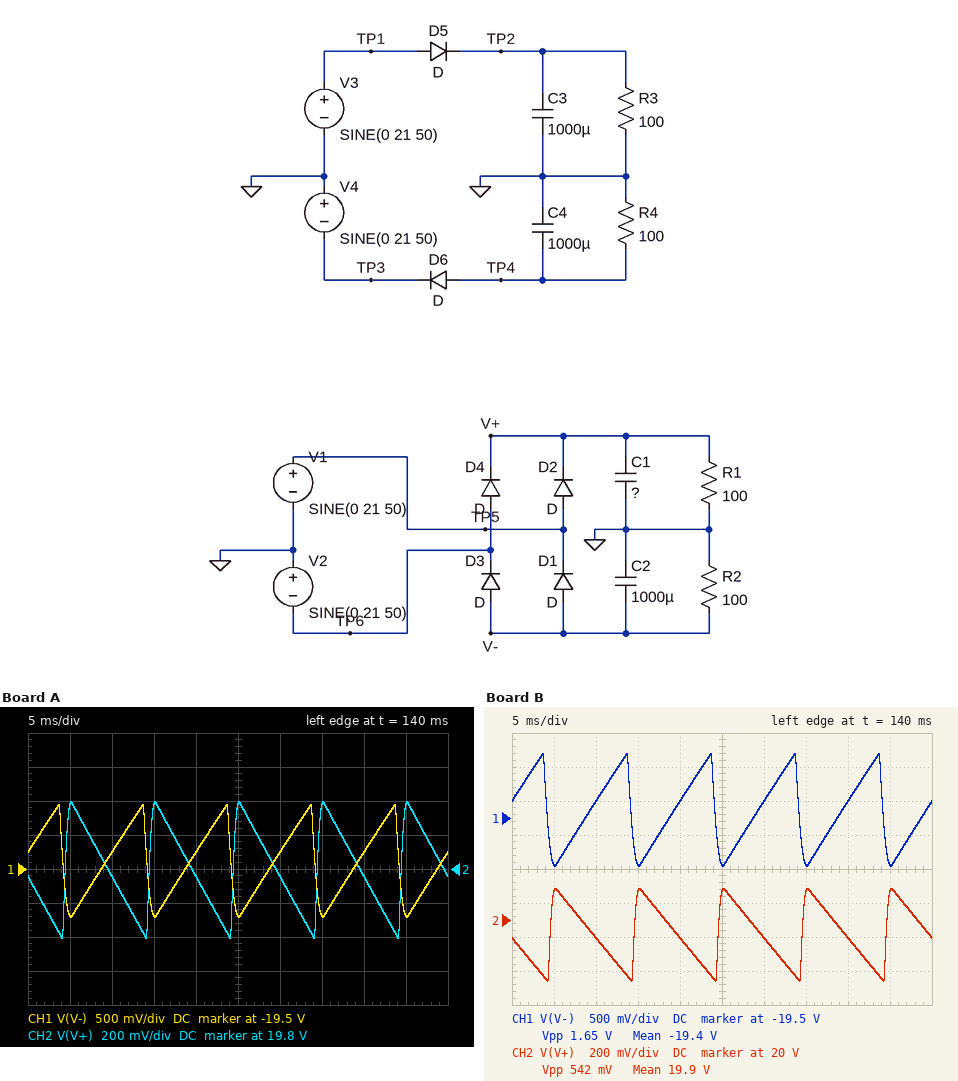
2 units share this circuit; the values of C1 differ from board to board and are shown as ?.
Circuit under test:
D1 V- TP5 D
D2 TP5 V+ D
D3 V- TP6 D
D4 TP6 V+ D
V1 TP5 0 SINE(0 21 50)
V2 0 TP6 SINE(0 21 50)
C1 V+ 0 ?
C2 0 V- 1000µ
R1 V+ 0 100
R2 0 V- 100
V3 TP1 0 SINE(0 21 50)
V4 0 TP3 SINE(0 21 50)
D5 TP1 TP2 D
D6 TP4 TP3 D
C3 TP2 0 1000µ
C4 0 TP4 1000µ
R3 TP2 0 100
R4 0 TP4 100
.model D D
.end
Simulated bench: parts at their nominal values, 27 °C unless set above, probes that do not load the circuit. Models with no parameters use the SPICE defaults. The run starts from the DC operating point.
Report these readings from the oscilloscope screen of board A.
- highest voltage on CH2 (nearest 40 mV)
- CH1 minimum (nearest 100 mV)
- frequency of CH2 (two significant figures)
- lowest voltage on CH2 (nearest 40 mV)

20.20 V
-20.2 V
100 Hz
19.40 V
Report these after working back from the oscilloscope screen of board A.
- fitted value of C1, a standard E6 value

2.2 mF
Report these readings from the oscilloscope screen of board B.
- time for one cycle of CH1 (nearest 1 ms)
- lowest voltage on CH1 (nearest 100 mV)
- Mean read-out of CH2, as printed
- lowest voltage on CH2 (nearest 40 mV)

10 ms
-20.2 V
19.9 V
19.64 V
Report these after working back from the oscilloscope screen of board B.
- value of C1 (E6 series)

3.3 mF
